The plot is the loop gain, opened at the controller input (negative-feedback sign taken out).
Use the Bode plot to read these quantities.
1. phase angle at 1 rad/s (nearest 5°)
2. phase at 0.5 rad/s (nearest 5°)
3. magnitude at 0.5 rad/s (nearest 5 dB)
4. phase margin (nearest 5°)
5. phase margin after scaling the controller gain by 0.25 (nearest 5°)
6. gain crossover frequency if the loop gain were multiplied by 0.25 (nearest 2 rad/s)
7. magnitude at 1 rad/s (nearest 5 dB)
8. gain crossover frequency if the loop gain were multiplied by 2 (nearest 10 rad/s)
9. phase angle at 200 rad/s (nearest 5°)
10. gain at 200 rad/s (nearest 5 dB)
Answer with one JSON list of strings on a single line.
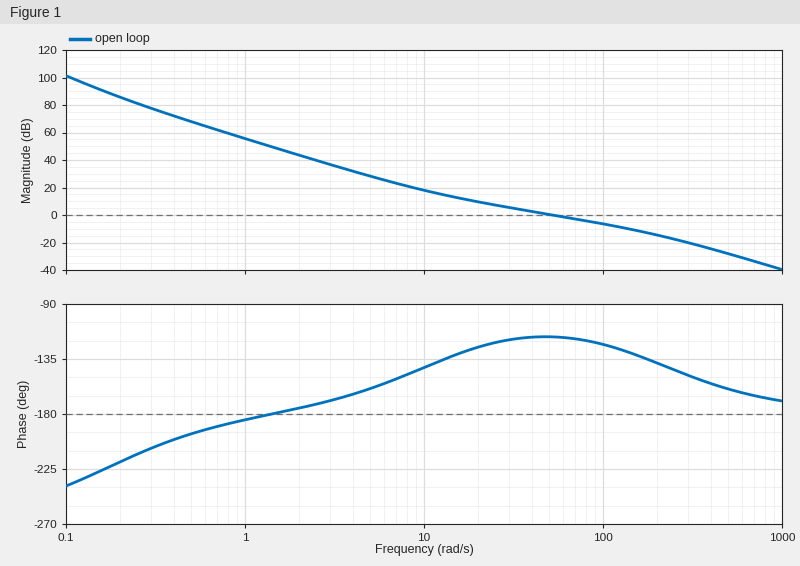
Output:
["-185°", "-195°", "70 dB", "65°", "50°", "16 rad/s", "55 dB", "100 rad/s", "-140°", "-15 dB"]
